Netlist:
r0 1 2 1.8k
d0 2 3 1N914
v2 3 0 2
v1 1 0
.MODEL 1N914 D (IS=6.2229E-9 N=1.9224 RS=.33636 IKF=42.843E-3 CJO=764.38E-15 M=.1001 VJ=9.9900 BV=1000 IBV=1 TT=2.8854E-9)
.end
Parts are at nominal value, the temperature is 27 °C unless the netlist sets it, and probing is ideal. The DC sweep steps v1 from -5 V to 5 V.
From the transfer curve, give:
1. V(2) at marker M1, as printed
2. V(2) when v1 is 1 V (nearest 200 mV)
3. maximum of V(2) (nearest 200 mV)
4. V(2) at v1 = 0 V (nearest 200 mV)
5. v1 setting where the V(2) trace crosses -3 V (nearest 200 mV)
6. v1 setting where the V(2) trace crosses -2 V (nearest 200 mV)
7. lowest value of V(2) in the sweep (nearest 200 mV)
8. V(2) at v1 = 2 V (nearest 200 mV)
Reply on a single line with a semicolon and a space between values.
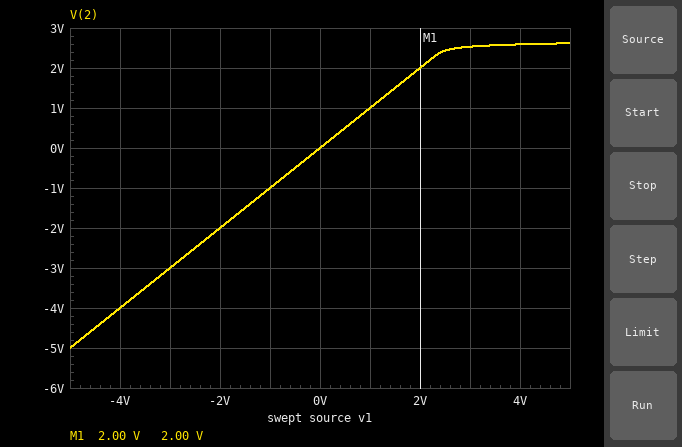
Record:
2.00 V; 1.0 V; 2.6 V; 0 V; -3.0 V; -2.0 V; -5.0 V; 2.0 V
